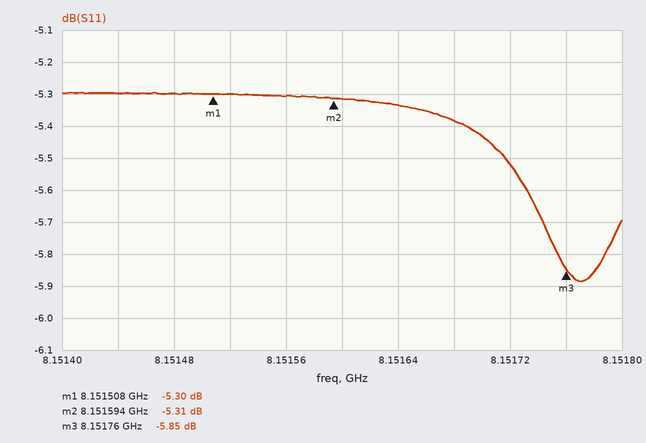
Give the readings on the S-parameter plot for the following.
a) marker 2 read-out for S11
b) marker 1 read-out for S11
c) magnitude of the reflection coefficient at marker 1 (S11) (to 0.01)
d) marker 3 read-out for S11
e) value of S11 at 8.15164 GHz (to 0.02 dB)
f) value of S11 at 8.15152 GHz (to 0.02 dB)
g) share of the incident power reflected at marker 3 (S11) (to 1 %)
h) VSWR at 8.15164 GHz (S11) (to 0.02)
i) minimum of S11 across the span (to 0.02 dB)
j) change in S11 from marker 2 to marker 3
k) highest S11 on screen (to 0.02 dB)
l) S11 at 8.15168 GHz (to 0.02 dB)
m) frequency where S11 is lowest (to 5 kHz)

-5.31 dB
-5.30 dB
0.54
-5.85 dB
-5.34 dB
-5.30 dB
26 %
3.36
-5.88 dB
-0.54 dB
-5.30 dB
-5.38 dB
8.151770 GHz
